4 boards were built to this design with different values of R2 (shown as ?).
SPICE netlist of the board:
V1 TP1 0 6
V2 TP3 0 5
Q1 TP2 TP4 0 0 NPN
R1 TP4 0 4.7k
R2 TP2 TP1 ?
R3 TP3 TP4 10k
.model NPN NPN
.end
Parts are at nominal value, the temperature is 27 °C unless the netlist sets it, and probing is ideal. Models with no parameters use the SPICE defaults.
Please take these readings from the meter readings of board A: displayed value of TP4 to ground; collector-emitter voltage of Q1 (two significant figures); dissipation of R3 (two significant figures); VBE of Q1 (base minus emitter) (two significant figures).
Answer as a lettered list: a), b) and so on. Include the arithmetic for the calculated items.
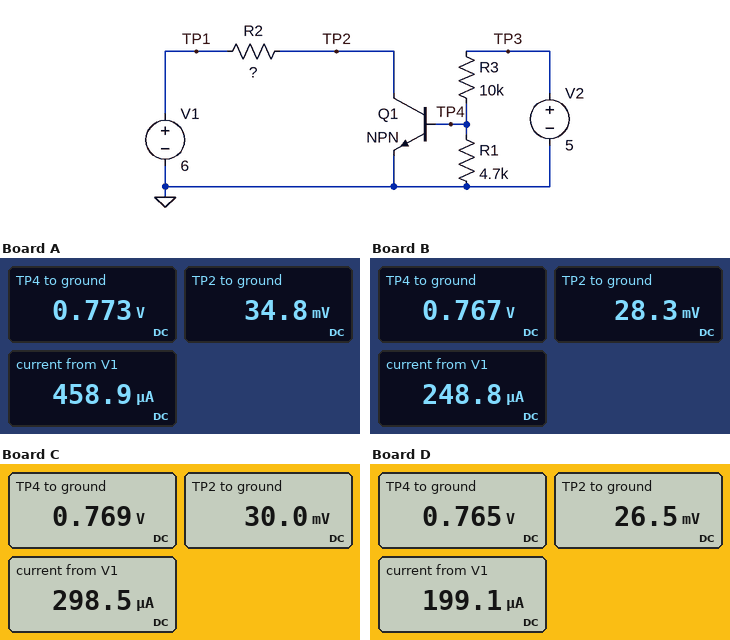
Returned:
a) 0.773 V
b) 34.8 mV = 35 mV
c) (5 V - 773 mV)^2 / 10 kΩ = 1.8 mW
d) 773 mV = 770 mV
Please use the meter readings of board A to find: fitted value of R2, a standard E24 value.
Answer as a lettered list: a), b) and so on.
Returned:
a) 13 kΩ
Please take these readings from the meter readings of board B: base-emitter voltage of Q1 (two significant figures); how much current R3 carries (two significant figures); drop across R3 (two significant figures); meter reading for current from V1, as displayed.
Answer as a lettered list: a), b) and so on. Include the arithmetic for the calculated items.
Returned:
a) 767 mV = 770 mV
b) (5 V - 767 mV) / 10 kΩ = 420 µA
c) 5 V - 767 mV = 4.2 V
d) 248.8 µA
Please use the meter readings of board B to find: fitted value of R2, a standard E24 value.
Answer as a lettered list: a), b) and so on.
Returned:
a) 24 kΩ
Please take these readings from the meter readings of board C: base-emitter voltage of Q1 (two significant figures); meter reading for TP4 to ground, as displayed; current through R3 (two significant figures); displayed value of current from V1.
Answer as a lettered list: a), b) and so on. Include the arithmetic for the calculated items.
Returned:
a) 769 mV = 770 mV
b) 0.769 V
c) (5 V - 769 mV) / 10 kΩ = 420 µA
d) 298.5 µA
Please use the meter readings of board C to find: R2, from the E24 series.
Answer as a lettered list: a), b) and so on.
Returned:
a) 20 kΩ
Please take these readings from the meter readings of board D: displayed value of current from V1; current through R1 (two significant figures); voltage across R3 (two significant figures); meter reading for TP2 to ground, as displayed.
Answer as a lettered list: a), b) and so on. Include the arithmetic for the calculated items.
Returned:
a) 199.1 µA
b) (765 mV) / 4.7 kΩ = 160 µA
c) 5 V - 765 mV = 4.2 V
d) 26.5 mV
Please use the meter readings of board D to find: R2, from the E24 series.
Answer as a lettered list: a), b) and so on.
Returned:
a) 30 kΩ
